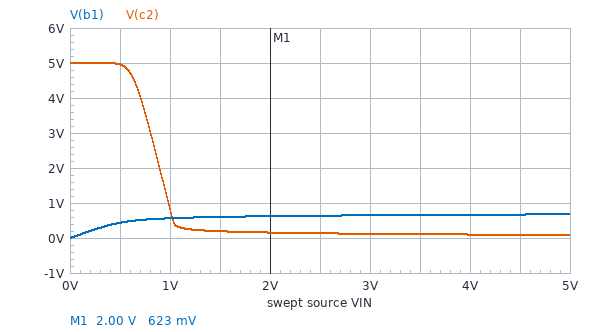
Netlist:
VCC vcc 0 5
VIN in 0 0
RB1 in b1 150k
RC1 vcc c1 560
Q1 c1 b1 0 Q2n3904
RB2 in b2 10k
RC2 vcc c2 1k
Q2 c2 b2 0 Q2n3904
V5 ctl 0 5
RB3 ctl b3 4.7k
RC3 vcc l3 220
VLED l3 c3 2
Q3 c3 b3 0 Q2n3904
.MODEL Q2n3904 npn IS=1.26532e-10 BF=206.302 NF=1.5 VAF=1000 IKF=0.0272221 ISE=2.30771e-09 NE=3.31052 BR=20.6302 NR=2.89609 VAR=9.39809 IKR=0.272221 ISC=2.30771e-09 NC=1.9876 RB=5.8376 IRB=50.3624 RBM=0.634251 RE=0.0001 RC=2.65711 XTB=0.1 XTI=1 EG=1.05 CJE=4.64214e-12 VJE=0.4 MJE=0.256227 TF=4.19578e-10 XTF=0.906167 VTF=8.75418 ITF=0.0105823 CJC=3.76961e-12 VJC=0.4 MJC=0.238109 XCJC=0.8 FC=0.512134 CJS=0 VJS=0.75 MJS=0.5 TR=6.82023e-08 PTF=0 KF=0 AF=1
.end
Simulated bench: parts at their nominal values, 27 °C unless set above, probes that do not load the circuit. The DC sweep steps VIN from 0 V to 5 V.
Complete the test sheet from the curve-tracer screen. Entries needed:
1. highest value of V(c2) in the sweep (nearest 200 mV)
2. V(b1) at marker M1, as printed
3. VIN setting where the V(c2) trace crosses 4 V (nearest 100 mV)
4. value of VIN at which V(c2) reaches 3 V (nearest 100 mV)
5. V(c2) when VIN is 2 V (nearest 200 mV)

5.0 V
623 mV
700 mV
800 mV
200 mV
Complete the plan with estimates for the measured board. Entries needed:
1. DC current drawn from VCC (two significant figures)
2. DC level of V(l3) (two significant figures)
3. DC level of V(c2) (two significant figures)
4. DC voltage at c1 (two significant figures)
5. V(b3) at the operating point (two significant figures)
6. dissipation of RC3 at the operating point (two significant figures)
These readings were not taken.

13 mA
2.1 V
5.0 V
5.0 V
740 mV
38 mW
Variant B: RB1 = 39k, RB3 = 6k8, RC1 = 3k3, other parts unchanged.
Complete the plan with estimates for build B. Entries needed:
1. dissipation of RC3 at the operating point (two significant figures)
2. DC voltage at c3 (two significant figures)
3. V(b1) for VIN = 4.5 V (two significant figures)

37 mW
140 mV
640 mV
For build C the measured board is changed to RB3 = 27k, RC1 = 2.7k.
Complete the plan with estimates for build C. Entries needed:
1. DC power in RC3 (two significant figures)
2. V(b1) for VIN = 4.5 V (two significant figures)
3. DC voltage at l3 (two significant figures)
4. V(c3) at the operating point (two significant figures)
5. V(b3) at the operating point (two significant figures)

34 mW
640 mV
2.3 V
260 mV
730 mV
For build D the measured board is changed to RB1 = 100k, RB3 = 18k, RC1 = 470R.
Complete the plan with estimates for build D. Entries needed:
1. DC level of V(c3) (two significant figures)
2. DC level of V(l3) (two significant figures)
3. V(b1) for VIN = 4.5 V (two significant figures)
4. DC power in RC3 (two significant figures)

210 mV
2.2 V
690 mV
35 mW
